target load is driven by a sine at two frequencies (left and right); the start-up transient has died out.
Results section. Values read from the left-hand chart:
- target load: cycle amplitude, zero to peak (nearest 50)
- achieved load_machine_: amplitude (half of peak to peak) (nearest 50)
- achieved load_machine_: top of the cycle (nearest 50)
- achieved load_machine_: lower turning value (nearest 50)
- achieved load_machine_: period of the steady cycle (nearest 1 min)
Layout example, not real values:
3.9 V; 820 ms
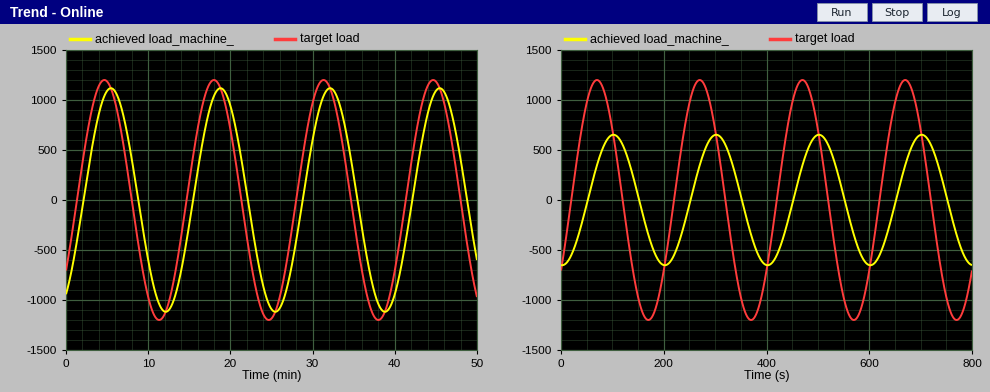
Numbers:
1200; 1100; 1100; -1100; 13 min
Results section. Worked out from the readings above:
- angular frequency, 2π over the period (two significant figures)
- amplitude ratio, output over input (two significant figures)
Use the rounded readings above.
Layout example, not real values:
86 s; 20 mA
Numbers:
0.48 rad/min; 0.92
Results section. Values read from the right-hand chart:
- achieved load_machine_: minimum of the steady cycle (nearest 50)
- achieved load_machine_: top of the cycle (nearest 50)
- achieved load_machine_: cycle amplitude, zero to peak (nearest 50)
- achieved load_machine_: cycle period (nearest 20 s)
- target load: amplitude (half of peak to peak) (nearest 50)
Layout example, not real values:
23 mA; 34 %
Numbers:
-650; 650; 650; 200 s; 1200
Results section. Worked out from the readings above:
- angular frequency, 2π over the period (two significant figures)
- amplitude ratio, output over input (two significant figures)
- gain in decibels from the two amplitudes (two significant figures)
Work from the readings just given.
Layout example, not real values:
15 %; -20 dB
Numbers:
0.031 rad/s; 0.54; -5.3 dB
